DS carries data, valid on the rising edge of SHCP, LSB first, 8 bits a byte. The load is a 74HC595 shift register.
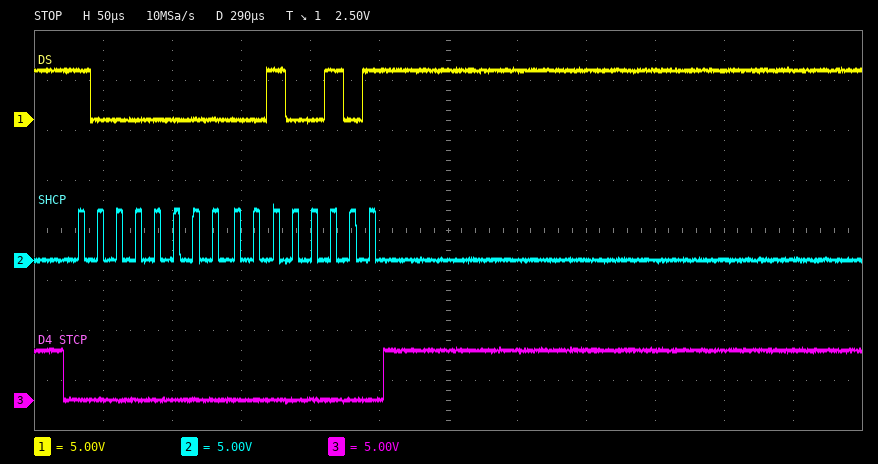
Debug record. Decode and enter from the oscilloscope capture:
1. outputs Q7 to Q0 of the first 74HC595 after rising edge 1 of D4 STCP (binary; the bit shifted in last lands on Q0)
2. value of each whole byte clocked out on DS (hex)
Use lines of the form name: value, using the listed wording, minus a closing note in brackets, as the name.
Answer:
outputs Q7 to Q0 of the first 74HC595 after rising edge 1 of D4 STCP: 00100101
value of each whole byte clocked out on DS: 01 A4
